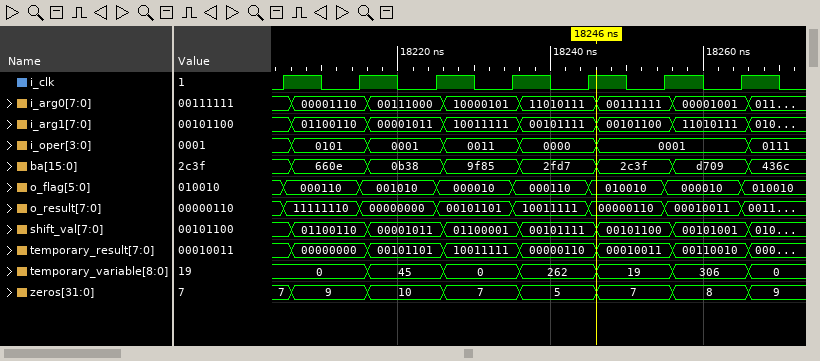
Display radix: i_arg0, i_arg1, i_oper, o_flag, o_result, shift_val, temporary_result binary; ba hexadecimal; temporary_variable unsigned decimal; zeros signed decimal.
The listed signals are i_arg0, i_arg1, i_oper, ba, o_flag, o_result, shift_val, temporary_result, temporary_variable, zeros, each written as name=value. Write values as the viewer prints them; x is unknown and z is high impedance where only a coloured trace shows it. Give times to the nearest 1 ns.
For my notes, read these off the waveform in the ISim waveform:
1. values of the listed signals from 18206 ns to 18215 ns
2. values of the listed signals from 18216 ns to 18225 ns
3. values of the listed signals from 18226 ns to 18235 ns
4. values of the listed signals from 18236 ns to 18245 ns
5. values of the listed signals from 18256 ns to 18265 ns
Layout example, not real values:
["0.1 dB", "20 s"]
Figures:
["i_arg0=00001110, i_arg1=01100110, i_oper=0101, ba=660e, o_flag=000110, o_result=11111110, shift_val=01100110, temporary_result=00000000, temporary_variable=0, zeros=9", "i_arg0=00111000, i_arg1=00001011, i_oper=0001, ba=0b38, o_flag=001010, o_result=00000000, shift_val=00001011, temporary_result=00101101, temporary_variable=45, zeros=10", "i_arg0=10000101, i_arg1=10011111, i_oper=0011, ba=9f85, o_flag=000010, o_result=00101101, shift_val=01100001, temporary_result=10011111, temporary_variable=0, zeros=7", "i_arg0=11010111, i_arg1=00101111, i_oper=0000, ba=2fd7, o_flag=000110, o_result=10011111, shift_val=00101111, temporary_result=00000110, temporary_variable=262, zeros=5", "i_arg0=00001001, i_arg1=11010111, i_oper=0001, ba=d709, o_flag=000010, o_result=00010011, shift_val=00101001, temporary_result=00110010, temporary_variable=306, zeros=8"]
